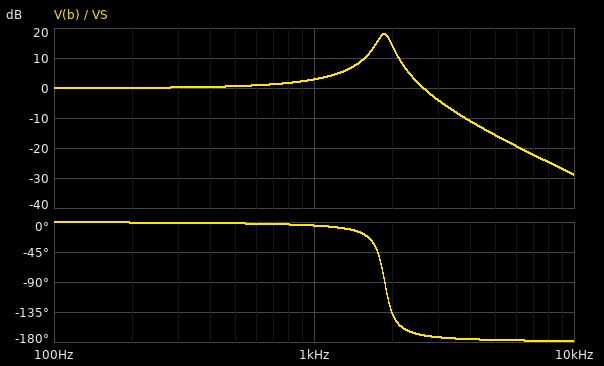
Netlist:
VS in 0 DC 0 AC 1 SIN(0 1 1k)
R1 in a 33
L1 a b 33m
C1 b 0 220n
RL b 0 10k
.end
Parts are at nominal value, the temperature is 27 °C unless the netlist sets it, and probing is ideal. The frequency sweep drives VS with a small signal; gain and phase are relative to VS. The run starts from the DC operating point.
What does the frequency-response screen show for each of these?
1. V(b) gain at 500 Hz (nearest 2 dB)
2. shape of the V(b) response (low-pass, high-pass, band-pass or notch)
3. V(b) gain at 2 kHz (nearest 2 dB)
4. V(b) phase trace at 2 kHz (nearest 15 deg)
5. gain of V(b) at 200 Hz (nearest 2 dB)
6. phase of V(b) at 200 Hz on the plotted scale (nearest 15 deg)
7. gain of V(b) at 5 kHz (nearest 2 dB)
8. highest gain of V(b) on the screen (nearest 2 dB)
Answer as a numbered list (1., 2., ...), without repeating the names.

1. 0 dB
2. low-pass
3. 14 dB
4. -135 deg
5. 0 dB
6. 0 deg
7. -16 dB
8. 18 dB
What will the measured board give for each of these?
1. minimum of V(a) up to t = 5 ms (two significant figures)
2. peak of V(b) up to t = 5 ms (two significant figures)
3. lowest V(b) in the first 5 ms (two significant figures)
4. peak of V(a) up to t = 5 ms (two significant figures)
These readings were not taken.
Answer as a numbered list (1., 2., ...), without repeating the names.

1. -1.0 V
2. 1.6 V
3. -1.7 V
4. 1.0 V
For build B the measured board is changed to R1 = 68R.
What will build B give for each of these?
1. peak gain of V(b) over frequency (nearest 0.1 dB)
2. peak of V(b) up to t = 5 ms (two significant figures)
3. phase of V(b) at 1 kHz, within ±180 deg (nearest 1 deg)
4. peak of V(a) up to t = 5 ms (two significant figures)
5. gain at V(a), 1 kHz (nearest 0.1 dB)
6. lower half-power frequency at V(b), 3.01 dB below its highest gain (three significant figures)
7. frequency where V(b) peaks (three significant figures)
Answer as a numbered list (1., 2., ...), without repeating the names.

1. 13.4 dB
2. 1.5 V
3. -9 deg
4. 980 mV
5. -0.2 dB
6. 1.64 kHz
7. 1.85 kHz
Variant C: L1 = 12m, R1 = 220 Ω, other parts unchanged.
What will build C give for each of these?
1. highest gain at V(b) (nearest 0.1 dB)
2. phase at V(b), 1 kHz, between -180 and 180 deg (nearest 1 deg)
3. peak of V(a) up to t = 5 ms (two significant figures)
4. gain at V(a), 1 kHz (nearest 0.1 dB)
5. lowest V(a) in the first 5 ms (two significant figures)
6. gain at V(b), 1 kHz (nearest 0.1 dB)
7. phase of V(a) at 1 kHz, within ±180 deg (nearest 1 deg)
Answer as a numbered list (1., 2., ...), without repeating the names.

1. 1.3 dB
2. -19 deg
3. 920 mV
4. -0.7 dB
5. -920 mV
6. 0.3 dB
7. -18 deg
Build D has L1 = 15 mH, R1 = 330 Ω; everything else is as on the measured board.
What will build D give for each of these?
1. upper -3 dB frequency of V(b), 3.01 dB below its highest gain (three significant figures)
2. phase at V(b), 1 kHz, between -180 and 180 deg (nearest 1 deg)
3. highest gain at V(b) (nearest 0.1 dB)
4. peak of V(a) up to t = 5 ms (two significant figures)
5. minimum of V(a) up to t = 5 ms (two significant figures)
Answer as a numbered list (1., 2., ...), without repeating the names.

1. 3.05 kHz
2. -27 deg
3. -0.1 dB
4. 860 mV
5. -860 mV
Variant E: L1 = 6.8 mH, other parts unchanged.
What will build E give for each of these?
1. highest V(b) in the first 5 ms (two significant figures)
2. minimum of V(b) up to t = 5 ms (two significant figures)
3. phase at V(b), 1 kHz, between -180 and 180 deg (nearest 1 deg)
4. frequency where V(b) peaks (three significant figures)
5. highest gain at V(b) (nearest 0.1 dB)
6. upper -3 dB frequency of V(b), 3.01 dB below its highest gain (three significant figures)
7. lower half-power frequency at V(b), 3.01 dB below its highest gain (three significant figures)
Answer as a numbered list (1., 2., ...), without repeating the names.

1. 1.1 V
2. -1.1 V
3. -3 deg
4. 4.08 kHz
5. 13.8 dB
6. 4.48 kHz
7. 3.63 kHz
